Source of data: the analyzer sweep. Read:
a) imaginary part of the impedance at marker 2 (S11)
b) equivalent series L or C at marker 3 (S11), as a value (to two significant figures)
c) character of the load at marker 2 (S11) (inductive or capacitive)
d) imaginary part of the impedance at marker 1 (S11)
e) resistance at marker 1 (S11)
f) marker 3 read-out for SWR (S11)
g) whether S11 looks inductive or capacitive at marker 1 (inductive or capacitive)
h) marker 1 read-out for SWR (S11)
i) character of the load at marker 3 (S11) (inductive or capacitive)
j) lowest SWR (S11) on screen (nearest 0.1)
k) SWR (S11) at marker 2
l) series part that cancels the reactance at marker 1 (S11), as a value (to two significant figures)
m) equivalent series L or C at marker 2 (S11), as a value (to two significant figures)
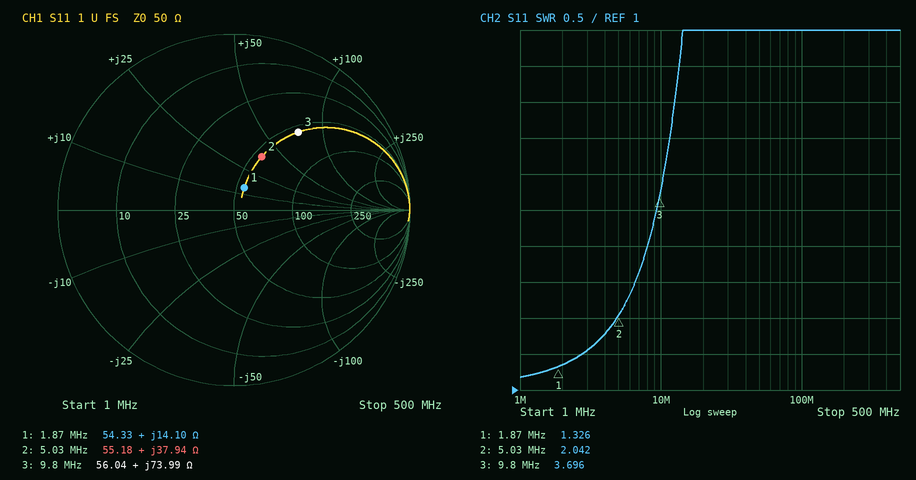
+37.94 Ω
1.2 µH
inductive
+14.10 Ω
54.33 Ω
3.696
inductive
1.326
inductive
1.2
2.042
6.0 nF
1.2 µH
